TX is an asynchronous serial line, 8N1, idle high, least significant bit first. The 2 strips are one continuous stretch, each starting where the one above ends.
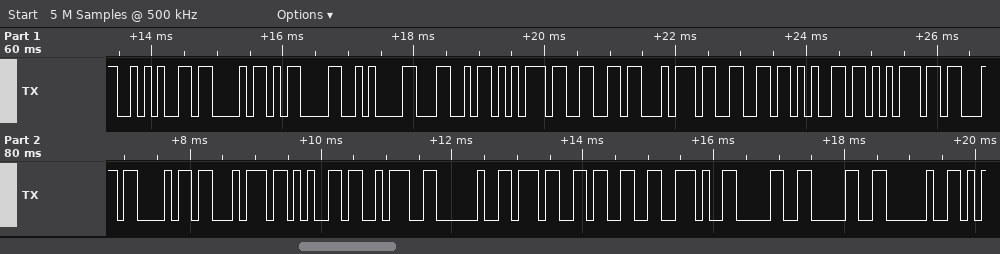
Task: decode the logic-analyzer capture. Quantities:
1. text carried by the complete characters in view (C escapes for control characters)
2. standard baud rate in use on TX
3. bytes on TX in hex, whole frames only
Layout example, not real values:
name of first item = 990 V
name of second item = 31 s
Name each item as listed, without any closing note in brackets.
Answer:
text carried by the complete characters in view = "*C\r\nLuftfeuchte: 73.00 "
standard baud rate in use on TX = 9600 baud
bytes on TX in hex, whole frames only = 2A 43 0D 0A 4C 75 66 74 66 65 75 63 68 74 65 3A 20 37 33 2E 30 30 20
